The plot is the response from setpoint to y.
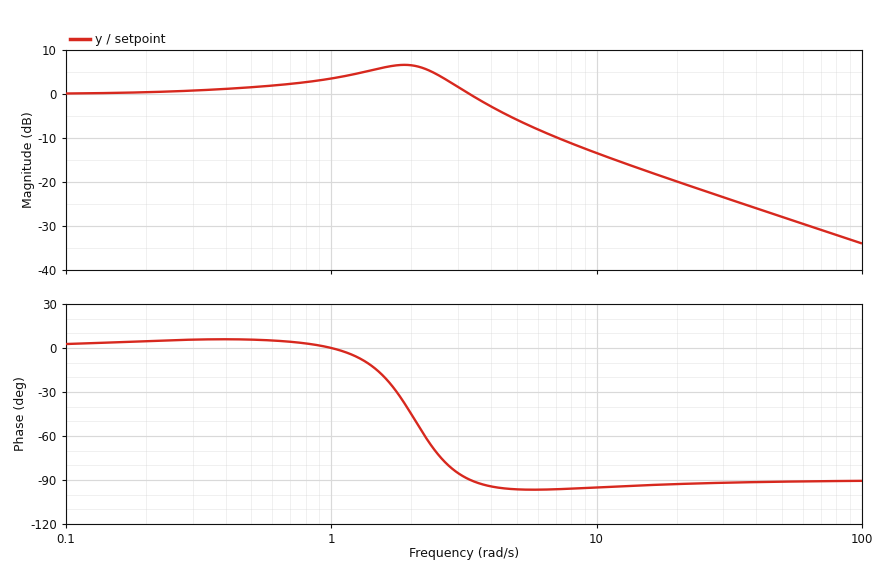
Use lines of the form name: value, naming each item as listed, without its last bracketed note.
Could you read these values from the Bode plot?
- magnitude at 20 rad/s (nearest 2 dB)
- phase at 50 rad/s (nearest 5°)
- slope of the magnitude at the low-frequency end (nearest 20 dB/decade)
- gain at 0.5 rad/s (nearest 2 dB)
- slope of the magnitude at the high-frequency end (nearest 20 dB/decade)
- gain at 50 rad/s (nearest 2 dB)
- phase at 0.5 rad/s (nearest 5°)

magnitude at 20 rad/s: -20 dB
phase at 50 rad/s: -90°
slope of the magnitude at the low-frequency end: 0 dB/decade
gain at 0.5 rad/s: 2 dB
slope of the magnitude at the high-frequency end: -20 dB/decade
gain at 50 rad/s: -28 dB
phase at 0.5 rad/s: 5°
